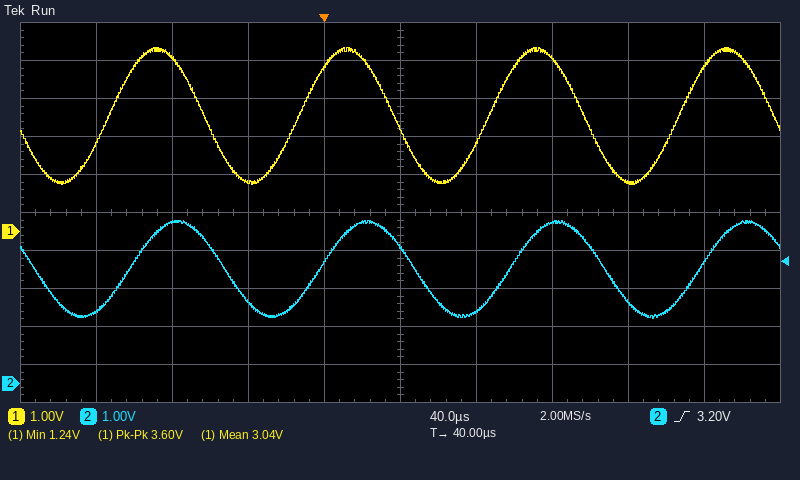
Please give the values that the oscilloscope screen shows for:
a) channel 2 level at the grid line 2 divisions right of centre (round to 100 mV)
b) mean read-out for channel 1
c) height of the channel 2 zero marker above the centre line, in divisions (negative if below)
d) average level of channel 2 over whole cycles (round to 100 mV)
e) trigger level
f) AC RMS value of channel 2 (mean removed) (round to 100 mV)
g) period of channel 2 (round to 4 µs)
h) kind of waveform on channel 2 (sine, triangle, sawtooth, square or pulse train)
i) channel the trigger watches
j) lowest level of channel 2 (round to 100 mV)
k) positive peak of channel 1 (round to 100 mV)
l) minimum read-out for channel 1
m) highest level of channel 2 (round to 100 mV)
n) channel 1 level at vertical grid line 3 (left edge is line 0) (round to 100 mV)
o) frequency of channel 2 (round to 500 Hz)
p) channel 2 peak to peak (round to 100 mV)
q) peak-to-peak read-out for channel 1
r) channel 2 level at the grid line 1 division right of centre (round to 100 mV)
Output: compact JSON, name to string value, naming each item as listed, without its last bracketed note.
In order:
{"channel 2 level at the grid line 2 divisions right of centre": "4.2 V", "mean read-out for channel 1": "3.04 V", "height of the channel 2 zero marker above the centre line, in divisions": "-4.5 div", "average level of channel 2 over whole cycles": "3.0 V", "trigger level": "3.20 V", "AC RMS value of channel 2 (mean removed)": "900 mV", "period of channel 2": "100 µs", "kind of waveform on channel 2": "sine", "channel the trigger watches": "channel 2", "lowest level of channel 2": "1.7 V", "positive peak of channel 1": "4.8 V", "minimum read-out for channel 1": "1.24 V", "highest level of channel 2": "4.3 V", "channel 1 level at vertical grid line 3 (left edge is line 0)": "1.3 V", "frequency of channel 2": "10.0 kHz", "channel 2 peak to peak": "2.6 V", "peak-to-peak read-out for channel 1": "3.60 V", "channel 2 level at the grid line 1 division right of centre": "1.9 V"}
